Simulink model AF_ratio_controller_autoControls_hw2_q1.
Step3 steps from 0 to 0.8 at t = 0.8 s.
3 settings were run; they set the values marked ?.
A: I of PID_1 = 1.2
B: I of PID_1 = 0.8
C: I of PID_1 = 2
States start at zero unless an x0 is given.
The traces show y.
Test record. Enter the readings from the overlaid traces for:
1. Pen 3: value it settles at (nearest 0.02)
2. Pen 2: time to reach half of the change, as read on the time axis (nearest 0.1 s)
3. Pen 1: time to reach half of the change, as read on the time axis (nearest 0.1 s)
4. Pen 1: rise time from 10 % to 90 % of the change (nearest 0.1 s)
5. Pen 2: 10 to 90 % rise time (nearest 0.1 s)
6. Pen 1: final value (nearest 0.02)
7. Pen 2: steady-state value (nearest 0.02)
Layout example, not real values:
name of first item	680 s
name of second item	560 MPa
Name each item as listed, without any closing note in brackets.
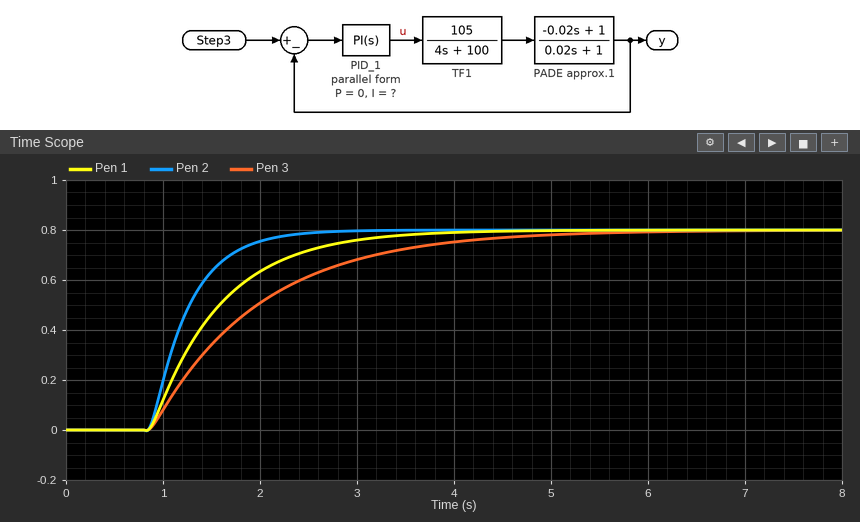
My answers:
Pen 3: value it settles at	0.80
Pen 2: time to reach half of the change, as read on the time axis	1.2 s
Pen 1: time to reach half of the change, as read on the time axis	1.4 s
Pen 1: rise time from 10 % to 90 % of the change	1.6 s
Pen 2: 10 to 90 % rise time	0.9 s
Pen 1: final value	0.80
Pen 2: steady-state value	0.80
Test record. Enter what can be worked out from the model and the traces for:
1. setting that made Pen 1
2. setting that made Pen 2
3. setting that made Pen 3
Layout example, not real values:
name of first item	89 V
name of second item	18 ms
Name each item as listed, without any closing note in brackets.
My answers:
setting that made Pen 1	A
setting that made Pen 2	C
setting that made Pen 3	B
